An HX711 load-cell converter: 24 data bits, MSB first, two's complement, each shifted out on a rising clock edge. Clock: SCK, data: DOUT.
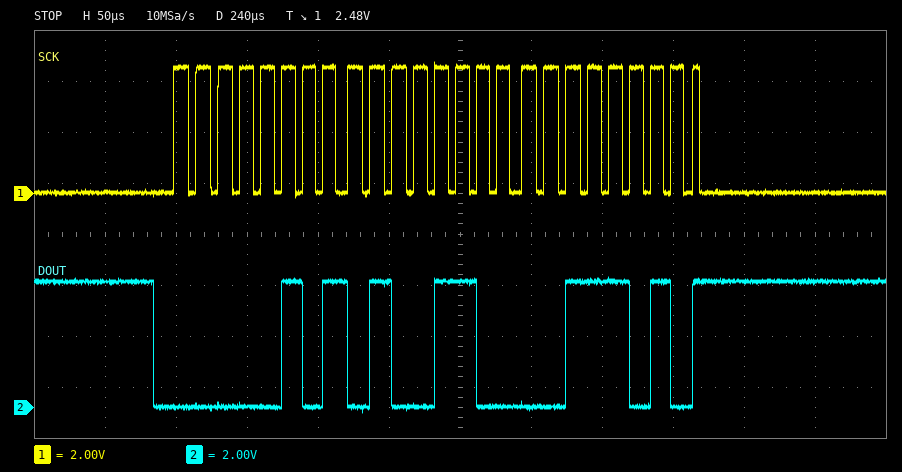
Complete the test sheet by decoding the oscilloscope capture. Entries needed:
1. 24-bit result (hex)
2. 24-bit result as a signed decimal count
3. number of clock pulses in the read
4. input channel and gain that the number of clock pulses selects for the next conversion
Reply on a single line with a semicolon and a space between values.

0x054C3A; 347194; 25; channel A, gain 128
